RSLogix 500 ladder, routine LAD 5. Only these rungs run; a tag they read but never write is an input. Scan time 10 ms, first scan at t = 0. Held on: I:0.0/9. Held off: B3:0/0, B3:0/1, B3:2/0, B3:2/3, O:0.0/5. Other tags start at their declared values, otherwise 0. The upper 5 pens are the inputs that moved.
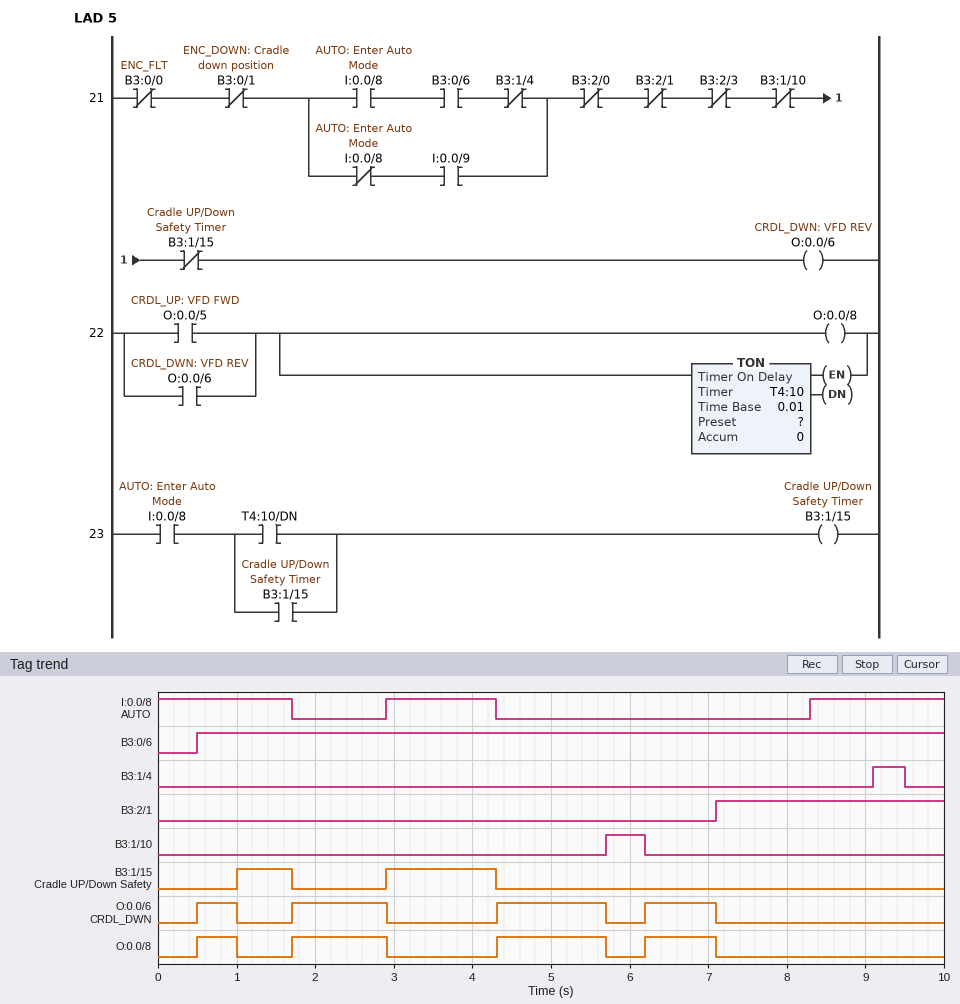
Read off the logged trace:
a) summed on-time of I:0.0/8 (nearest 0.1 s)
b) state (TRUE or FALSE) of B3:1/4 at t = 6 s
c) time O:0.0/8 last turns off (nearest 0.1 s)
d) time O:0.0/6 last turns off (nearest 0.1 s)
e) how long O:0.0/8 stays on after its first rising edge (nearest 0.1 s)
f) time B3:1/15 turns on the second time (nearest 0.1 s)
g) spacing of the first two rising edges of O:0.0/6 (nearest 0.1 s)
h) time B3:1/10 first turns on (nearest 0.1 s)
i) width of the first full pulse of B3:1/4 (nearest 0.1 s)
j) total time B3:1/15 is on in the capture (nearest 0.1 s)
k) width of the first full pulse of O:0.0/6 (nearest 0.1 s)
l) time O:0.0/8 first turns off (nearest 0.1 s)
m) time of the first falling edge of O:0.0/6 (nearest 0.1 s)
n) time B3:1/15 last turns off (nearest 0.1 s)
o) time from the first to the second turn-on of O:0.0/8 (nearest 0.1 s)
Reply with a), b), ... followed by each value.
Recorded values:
a) 4.8 s
b) FALSE
c) 7.1 s
d) 7.1 s
e) 0.5 s
f) 2.9 s
g) 1.2 s
h) 5.7 s
i) 0.4 s
j) 2.1 s
k) 0.5 s
l) 1.0 s
m) 1.0 s
n) 4.3 s
o) 1.2 s
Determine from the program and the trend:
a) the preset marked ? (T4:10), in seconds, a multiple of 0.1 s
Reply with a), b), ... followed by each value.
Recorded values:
a) 0.5 s
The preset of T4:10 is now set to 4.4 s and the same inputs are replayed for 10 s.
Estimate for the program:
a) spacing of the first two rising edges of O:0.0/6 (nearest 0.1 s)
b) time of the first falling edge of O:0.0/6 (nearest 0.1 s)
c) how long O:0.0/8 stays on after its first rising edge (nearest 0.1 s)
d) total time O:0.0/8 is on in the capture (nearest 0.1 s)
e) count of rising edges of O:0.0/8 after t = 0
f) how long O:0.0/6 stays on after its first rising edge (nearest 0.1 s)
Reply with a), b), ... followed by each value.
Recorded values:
a) 5.7 s
b) 5.7 s
c) 5.2 s
d) 6.1 s
e) 2
f) 5.2 s
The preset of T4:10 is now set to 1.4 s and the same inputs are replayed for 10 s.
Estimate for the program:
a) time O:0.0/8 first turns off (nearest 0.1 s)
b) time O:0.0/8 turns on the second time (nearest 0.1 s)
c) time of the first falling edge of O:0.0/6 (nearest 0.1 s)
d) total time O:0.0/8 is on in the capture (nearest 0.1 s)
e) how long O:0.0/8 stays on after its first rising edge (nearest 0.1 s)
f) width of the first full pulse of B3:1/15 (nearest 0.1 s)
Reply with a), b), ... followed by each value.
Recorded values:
a) 2.9 s
b) 4.3 s
c) 2.9 s
d) 4.7 s
e) 2.4 s
f) 1.4 s
